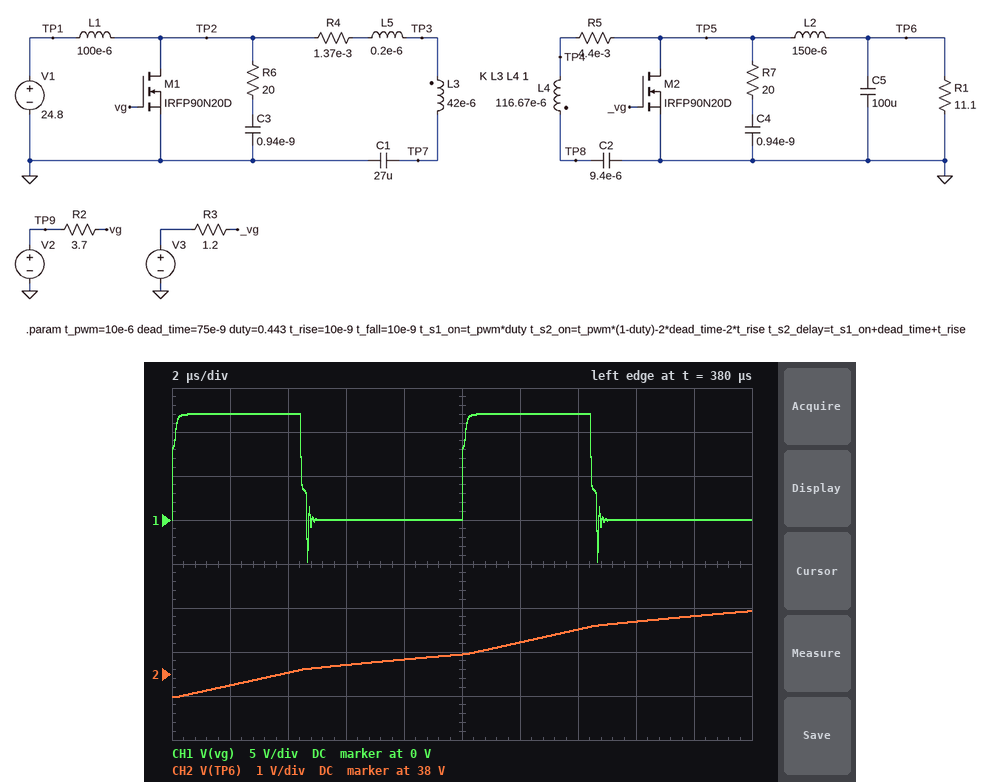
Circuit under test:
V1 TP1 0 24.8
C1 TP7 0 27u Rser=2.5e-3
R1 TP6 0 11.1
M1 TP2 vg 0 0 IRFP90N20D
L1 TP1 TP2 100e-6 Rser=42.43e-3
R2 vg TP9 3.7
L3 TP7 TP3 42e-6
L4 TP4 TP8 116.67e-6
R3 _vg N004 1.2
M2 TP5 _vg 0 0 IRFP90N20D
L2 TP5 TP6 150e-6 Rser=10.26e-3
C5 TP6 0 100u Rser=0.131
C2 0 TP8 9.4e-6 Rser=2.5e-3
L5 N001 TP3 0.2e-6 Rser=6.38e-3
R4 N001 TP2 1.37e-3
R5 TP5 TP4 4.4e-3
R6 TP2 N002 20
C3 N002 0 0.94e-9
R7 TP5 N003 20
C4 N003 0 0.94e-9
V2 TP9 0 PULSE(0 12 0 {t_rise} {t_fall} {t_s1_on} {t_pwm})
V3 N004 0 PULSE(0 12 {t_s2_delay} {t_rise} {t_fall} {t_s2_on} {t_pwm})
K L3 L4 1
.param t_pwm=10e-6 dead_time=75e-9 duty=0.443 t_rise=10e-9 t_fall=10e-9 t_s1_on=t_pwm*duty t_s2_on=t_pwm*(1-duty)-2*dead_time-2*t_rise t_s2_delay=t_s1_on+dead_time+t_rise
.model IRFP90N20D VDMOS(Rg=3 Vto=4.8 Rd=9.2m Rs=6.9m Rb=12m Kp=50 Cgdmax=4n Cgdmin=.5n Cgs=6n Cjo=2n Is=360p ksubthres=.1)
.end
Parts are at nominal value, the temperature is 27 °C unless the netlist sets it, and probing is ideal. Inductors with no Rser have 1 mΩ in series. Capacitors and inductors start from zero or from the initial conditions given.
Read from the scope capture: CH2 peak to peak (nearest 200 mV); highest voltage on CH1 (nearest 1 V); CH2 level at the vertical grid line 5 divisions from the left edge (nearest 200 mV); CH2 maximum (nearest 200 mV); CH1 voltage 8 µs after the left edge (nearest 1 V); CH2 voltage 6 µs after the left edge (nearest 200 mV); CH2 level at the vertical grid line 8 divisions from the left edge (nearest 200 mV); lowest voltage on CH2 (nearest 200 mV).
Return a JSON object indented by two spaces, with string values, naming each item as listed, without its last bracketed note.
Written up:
{
  "CH2 peak to peak": "2.0 V",
  "highest voltage on CH1": "12 V",
  "CH2 level at the vertical grid line 5 divisions from the left edge": "38.4 V",
  "CH2 maximum": "39.4 V",
  "CH1 voltage 8 µs after the left edge": "0 V",
  "CH2 voltage 6 µs after the left edge": "38.2 V",
  "CH2 level at the vertical grid line 8 divisions from the left edge": "39.2 V",
  "lowest voltage on CH2": "37.4 V"
}
